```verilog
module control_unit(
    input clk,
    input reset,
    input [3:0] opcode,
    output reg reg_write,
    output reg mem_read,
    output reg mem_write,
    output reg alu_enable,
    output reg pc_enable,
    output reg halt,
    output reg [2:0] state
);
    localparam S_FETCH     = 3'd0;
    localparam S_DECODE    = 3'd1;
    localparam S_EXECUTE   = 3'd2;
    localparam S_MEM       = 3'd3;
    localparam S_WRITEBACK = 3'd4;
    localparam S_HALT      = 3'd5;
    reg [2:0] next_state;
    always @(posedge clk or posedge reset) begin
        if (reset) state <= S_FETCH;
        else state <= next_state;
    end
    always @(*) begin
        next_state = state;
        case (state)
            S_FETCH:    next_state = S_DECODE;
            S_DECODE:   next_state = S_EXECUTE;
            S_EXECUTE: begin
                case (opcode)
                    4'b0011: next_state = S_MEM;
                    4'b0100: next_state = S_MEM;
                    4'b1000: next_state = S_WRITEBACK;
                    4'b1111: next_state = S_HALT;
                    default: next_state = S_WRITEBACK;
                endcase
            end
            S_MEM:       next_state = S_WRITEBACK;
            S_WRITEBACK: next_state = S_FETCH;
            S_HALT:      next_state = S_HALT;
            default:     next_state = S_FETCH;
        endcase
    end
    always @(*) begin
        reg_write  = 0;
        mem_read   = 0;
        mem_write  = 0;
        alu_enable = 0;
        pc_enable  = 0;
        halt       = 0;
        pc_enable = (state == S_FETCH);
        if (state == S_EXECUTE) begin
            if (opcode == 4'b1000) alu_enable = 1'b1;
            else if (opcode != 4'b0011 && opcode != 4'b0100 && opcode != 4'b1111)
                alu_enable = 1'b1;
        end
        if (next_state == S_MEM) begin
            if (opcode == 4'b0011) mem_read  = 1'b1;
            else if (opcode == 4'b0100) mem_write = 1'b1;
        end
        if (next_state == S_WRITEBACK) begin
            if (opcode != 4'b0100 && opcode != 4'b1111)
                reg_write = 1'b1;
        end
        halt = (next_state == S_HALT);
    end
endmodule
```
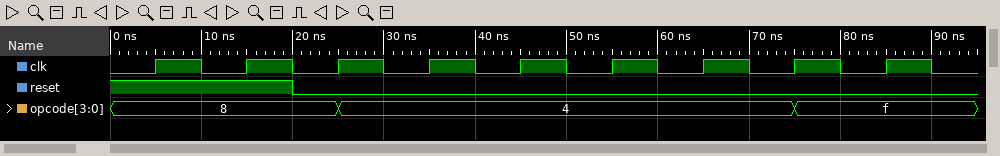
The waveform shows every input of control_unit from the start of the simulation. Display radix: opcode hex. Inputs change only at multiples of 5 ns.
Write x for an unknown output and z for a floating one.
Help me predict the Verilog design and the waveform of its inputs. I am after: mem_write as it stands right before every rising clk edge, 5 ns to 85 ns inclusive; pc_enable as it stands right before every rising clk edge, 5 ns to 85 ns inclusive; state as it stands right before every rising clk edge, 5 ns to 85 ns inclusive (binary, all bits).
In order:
0 0 0 0 1 0 0 0 0
1 1 1 0 0 0 0 1 0
000, 000, 000, 001, 010, 011, 100, 000, 001
